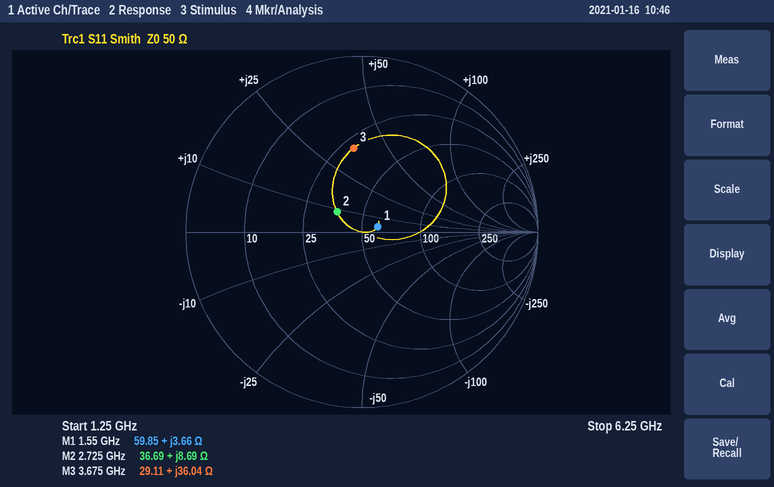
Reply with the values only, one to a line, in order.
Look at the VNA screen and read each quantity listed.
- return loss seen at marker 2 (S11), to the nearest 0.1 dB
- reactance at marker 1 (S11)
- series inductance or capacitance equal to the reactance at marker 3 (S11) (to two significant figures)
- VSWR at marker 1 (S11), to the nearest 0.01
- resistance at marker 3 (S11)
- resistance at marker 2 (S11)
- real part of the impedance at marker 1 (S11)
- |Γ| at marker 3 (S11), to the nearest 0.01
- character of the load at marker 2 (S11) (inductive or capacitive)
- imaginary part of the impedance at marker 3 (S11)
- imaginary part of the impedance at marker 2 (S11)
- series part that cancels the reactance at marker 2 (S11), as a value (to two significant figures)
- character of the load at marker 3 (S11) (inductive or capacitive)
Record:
14.8 dB
+3.66 Ω
1.6 nH
1.21
29.11 Ω
36.69 Ω
59.85 Ω
0.48
inductive
+36.04 Ω
+8.69 Ω
6.7 pF
inductive
